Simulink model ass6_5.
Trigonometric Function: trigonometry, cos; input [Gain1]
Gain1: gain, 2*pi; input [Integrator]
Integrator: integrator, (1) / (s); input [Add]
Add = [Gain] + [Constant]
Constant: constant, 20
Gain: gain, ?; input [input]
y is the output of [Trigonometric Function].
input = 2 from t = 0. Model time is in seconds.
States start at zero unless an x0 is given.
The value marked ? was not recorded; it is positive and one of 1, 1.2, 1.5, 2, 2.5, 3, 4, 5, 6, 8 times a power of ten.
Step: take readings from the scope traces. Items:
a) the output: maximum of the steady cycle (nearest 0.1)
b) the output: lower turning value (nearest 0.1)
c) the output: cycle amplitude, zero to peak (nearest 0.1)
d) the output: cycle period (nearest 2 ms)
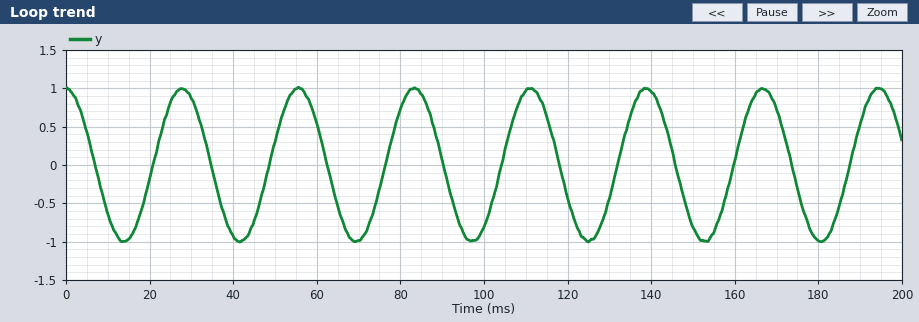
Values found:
1.0
-1.0
1.0
28 ms
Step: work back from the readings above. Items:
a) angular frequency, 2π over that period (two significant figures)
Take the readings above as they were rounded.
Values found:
0.22 rad/ms
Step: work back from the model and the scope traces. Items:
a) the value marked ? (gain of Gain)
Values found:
8
